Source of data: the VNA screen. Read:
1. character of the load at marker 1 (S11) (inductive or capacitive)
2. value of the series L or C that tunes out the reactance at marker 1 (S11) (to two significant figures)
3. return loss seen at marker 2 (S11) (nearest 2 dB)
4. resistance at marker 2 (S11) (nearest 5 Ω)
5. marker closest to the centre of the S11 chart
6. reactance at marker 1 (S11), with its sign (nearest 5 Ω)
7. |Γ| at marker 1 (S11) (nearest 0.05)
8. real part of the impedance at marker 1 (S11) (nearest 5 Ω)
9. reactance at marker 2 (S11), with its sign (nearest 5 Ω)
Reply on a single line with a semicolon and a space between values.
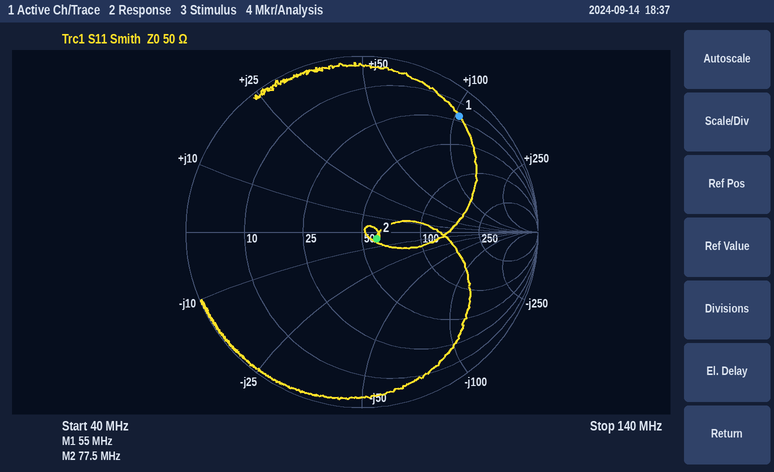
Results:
inductive; 28 pF; 20 dB; 60 Ω; marker 2; +105 Ω; 0.85; 20 Ω; -5 Ω
